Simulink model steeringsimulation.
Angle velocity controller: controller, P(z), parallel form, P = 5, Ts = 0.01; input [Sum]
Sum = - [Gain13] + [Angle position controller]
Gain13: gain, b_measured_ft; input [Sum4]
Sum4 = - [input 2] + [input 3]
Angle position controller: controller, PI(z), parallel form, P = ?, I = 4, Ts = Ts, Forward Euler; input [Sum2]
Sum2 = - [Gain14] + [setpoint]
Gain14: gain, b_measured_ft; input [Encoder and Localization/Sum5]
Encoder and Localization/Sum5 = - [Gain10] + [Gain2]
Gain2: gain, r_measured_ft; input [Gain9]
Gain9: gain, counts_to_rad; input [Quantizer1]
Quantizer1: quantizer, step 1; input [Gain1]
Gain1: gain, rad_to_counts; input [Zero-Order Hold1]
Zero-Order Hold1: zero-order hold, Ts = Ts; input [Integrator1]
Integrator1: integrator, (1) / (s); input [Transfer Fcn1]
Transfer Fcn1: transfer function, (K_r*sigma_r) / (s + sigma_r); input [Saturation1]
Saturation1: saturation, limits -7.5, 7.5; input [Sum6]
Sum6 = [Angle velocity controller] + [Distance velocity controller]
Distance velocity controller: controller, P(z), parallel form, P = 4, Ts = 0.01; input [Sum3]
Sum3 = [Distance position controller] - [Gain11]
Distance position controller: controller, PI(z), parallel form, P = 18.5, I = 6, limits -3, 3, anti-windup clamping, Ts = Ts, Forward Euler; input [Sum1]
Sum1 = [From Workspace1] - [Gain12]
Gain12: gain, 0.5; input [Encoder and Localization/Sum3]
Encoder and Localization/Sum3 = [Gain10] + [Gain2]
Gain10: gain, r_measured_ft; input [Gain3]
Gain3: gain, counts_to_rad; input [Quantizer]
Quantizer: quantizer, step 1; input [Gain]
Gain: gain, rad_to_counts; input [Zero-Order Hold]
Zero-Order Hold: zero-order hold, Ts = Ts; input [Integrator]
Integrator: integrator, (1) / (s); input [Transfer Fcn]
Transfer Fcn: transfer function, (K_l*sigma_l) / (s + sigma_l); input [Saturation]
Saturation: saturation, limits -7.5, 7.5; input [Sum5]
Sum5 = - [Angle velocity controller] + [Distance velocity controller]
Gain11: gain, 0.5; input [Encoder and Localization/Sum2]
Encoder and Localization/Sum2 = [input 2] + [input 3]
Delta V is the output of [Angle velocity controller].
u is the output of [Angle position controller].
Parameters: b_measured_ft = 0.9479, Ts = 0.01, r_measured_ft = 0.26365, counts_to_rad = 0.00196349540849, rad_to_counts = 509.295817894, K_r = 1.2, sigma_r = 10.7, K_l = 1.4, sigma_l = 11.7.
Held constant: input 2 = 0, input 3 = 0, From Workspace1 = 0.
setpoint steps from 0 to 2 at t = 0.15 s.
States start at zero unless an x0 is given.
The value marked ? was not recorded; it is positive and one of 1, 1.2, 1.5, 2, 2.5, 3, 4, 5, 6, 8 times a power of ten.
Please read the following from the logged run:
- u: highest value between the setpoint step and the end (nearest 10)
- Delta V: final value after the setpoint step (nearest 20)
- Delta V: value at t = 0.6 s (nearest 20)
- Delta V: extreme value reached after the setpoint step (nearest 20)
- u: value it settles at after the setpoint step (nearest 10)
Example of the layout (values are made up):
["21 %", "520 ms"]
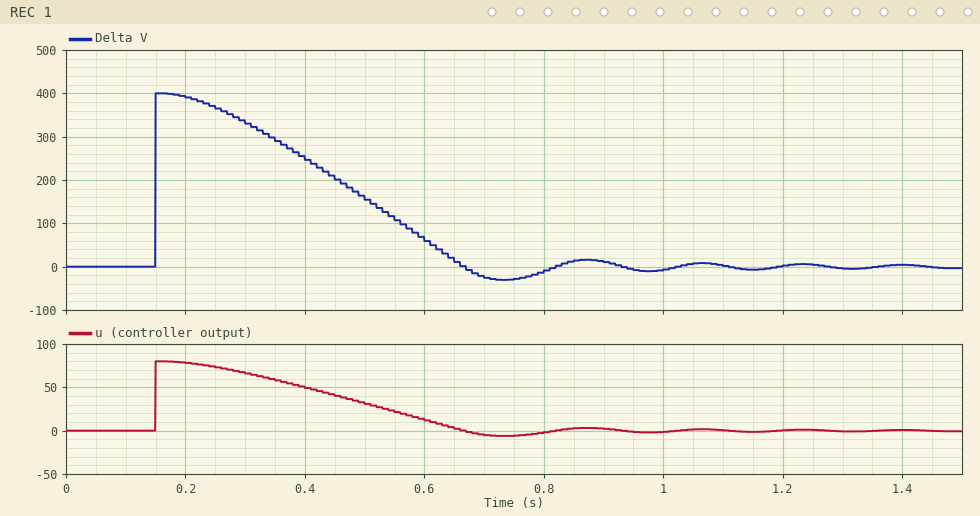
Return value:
["80", "0", "60", "400", "0"]
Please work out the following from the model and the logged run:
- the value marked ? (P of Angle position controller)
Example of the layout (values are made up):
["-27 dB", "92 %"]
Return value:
["40"]
